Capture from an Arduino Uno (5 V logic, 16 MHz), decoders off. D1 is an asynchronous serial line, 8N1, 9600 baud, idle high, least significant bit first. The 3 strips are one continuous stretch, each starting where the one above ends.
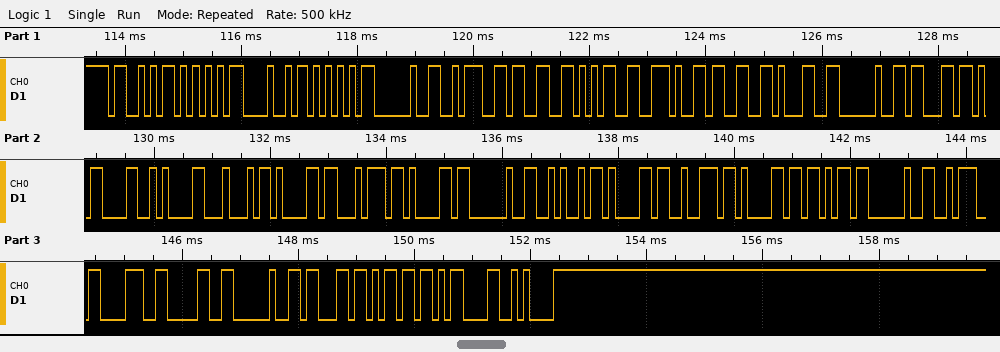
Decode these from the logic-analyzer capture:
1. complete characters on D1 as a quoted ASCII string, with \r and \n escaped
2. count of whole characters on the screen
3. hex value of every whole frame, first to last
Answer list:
"SUHU :35.31 c\r\nData Jarak :80 cm\r\n"
34
53 55 48 55 20 3A 33 35 2E 33 31 20 63 0D 0A 44 61 74 61 20 4A 61 72 61 6B 20 3A 38 30 20 63 6D 0D 0A
